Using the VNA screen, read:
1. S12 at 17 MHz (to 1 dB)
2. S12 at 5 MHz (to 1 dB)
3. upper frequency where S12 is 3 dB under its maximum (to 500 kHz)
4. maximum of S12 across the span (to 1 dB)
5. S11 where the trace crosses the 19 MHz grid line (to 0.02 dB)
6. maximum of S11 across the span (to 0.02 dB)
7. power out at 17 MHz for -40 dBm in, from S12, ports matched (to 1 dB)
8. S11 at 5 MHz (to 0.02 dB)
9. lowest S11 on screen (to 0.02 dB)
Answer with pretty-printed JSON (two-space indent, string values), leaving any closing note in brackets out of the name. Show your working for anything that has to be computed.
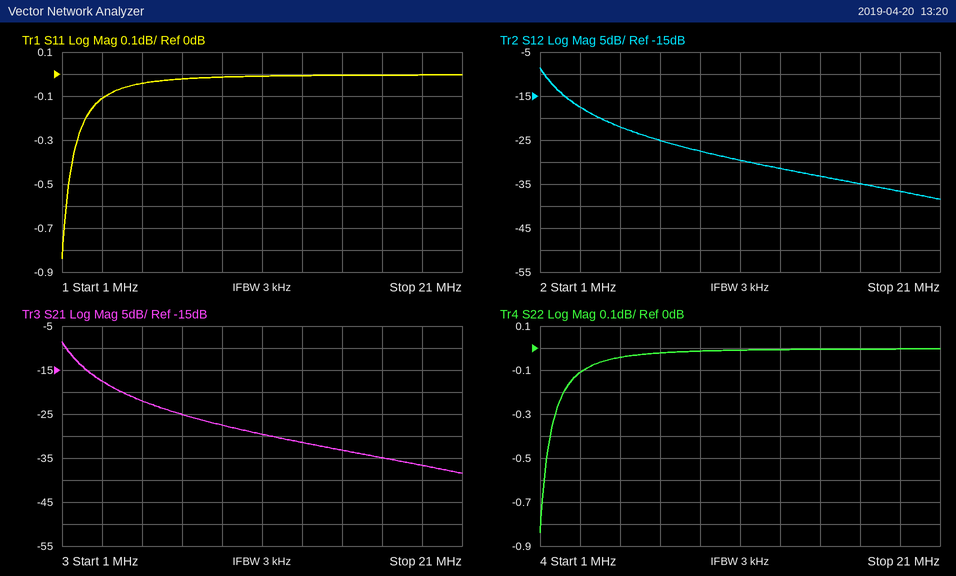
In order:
{
  "S12 at 17 MHz": "-35 dB",
  "S12 at 5 MHz": "-22 dB",
  "upper frequency where S12 is 3 dB under its maximum": "1.5 MHz",
  "maximum of S12 across the span": "-9 dB",
  "S11 where the trace crosses the 19 MHz grid line": "0.00 dB",
  "maximum of S11 across the span": "0.00 dB",
  "power out at 17 MHz for -40 dBm in, from S12, ports matched": "-40 dBm + (-35 dB) = -75 dBm",
  "S11 at 5 MHz": "-0.04 dB",
  "lowest S11 on screen": "-0.84 dB"
}
